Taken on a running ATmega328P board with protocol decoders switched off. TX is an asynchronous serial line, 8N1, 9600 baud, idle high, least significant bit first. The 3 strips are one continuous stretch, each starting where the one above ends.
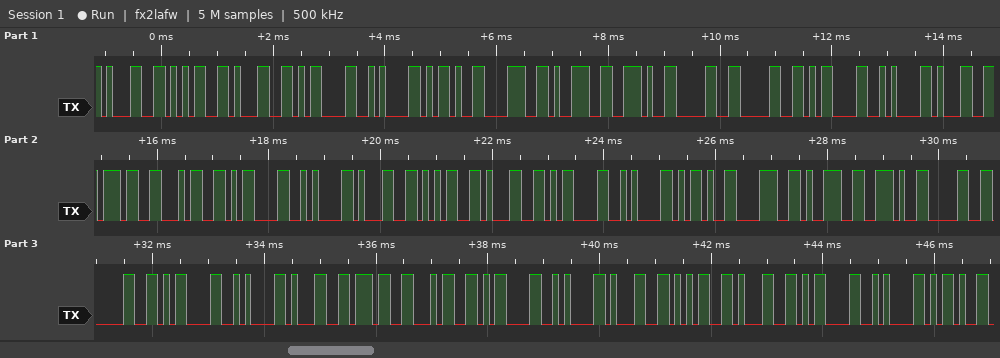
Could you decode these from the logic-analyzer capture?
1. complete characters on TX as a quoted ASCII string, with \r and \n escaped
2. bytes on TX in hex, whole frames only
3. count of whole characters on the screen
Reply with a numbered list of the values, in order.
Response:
1. "151\r\n-89.00\r\n174\r\n151\r\n-89.00\r\n174\r\n151\r\n-"
2. 31 35 31 0D 0A 2D 38 39 2E 30 30 0D 0A 31 37 34 0D 0A 31 35 31 0D 0A 2D 38 39 2E 30 30 0D 0A 31 37 34 0D 0A 31 35 31 0D 0A 2D
3. 42
